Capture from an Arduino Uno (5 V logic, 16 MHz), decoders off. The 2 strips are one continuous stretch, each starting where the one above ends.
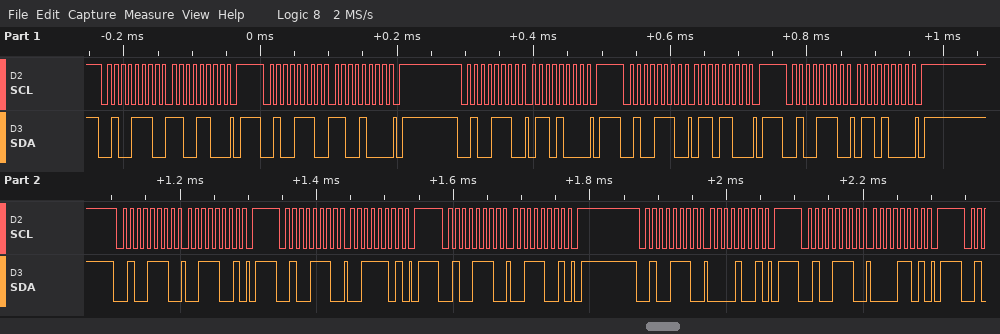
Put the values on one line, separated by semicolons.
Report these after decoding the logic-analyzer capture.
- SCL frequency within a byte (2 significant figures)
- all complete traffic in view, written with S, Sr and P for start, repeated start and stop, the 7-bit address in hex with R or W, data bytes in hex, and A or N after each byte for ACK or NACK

100 kHz; S 27W A CC A P S 27W A C8 A P S 27W A 68 A P S 27W A 6C A P S 27W A 68 A P S 27W A 39 A P S 27W A 3D A P S 27W A 39 A P S 27W A 09 A P S 27W A 0D A P
